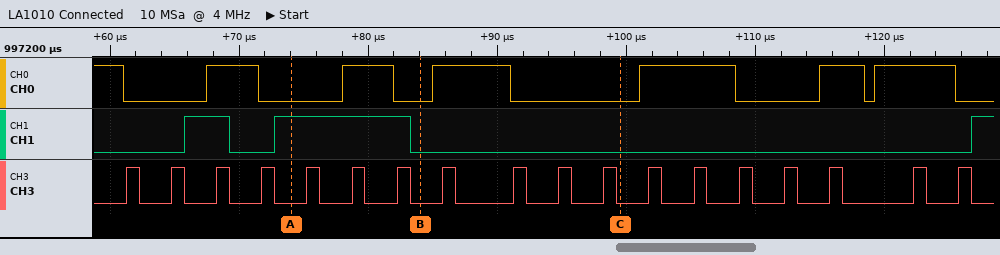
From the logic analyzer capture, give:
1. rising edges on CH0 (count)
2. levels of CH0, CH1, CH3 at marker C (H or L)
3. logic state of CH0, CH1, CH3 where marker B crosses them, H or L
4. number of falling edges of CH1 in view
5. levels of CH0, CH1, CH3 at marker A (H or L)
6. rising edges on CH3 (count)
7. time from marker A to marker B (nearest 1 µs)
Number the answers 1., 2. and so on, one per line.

1. 6
2. CH0=L, CH1=L, CH3=L
3. CH0=L, CH1=L, CH3=L
4. 2
5. CH0=L, CH1=H, CH3=L
6. 18
7. 10 µs
